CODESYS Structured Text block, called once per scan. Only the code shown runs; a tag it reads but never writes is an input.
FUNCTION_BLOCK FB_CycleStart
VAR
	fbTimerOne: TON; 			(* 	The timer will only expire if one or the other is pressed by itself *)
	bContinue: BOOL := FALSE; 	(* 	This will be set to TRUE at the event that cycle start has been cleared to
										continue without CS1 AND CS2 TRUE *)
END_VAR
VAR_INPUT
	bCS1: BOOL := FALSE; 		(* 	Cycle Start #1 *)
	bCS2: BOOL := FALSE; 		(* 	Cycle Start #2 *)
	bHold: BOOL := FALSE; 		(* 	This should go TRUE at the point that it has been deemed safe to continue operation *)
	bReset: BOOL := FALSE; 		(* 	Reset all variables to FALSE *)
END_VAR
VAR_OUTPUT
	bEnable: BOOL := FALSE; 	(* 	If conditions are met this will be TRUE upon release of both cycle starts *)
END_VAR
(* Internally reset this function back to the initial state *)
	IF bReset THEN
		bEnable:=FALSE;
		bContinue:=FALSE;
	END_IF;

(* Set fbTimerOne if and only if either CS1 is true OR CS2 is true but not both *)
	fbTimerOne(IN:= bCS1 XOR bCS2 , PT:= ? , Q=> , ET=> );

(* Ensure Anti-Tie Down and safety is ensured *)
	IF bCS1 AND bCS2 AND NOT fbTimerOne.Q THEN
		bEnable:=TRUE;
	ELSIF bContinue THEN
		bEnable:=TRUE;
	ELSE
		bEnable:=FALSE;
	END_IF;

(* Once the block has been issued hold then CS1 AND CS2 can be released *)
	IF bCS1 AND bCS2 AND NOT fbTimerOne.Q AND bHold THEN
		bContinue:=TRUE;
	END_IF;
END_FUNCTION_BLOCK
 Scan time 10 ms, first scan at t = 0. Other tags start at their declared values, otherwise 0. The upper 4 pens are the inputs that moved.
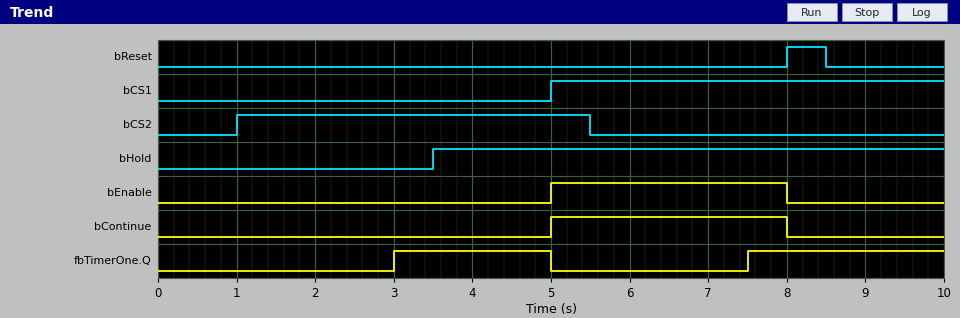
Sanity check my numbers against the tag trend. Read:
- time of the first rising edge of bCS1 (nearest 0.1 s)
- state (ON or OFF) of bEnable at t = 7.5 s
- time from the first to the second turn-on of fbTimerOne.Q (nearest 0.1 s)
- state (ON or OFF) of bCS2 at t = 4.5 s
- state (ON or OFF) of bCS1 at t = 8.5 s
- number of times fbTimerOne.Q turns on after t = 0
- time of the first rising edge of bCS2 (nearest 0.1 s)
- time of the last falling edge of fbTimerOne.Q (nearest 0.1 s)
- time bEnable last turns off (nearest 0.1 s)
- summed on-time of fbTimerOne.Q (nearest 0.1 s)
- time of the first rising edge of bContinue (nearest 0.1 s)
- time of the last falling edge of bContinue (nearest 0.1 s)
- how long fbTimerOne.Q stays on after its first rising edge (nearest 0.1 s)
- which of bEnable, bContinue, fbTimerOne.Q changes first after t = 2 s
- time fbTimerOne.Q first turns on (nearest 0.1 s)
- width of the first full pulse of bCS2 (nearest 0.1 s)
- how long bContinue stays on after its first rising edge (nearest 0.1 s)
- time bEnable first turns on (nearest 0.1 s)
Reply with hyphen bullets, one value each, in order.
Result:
- 5.0 s
- ON
- 4.5 s
- ON
- ON
- 2
- 1.0 s
- 5.0 s
- 8.0 s
- 4.5 s
- 5.0 s
- 8.0 s
- 2.0 s
- fbTimerOne.Q
- 3.0 s
- 4.5 s
- 3.0 s
- 5.0 s
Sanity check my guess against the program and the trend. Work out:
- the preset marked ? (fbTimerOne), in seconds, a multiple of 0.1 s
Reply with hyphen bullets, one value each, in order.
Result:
- 2.0 s
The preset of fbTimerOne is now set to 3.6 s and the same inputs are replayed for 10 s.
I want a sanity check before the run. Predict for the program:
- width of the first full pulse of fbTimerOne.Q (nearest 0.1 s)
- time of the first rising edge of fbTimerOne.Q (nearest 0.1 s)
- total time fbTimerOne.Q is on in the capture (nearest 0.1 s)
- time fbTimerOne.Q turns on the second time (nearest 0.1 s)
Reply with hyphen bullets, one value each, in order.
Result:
- 0.4 s
- 4.6 s
- 1.3 s
- 9.1 s
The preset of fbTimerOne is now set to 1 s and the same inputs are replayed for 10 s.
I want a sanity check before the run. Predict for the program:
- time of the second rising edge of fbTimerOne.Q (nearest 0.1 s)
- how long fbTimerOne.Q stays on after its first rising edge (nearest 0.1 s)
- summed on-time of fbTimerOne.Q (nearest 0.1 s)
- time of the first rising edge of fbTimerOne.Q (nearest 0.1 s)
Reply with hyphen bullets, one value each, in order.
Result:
- 6.5 s
- 3.0 s
- 6.5 s
- 2.0 s
